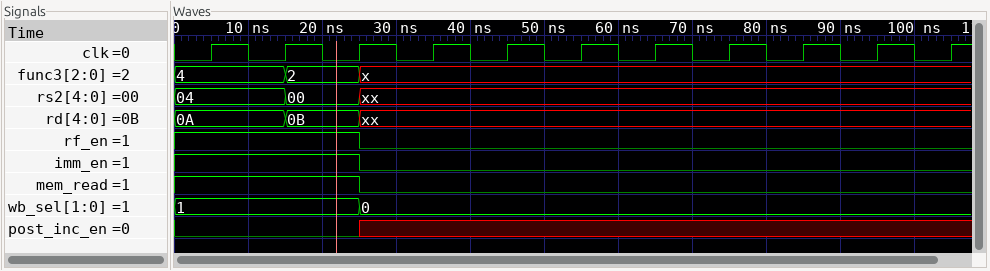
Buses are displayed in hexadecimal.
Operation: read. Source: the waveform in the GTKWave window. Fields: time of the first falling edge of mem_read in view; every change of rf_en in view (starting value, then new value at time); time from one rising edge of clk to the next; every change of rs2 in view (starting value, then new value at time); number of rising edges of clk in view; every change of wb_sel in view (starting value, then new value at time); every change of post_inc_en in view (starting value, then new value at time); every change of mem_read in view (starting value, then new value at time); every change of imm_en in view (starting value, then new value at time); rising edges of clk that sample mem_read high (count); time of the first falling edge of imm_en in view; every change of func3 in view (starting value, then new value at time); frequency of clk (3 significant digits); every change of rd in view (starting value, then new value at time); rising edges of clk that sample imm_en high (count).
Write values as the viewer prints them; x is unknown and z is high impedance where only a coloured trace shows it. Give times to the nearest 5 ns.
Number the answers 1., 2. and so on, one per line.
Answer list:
1. 25 ns
2. 1, 0 at 25 ns
3. 10 ns
4. 04, 00 at 15 ns, xx at 25 ns
5. 11
6. 1, 0 at 25 ns
7. 0, x at 25 ns
8. 1, 0 at 25 ns
9. 1, 0 at 25 ns
10. 3
11. 25 ns
12. 4, 2 at 15 ns, x at 25 ns
13. 100 MHz
14. 0A, 0B at 15 ns, xx at 25 ns
15. 3
